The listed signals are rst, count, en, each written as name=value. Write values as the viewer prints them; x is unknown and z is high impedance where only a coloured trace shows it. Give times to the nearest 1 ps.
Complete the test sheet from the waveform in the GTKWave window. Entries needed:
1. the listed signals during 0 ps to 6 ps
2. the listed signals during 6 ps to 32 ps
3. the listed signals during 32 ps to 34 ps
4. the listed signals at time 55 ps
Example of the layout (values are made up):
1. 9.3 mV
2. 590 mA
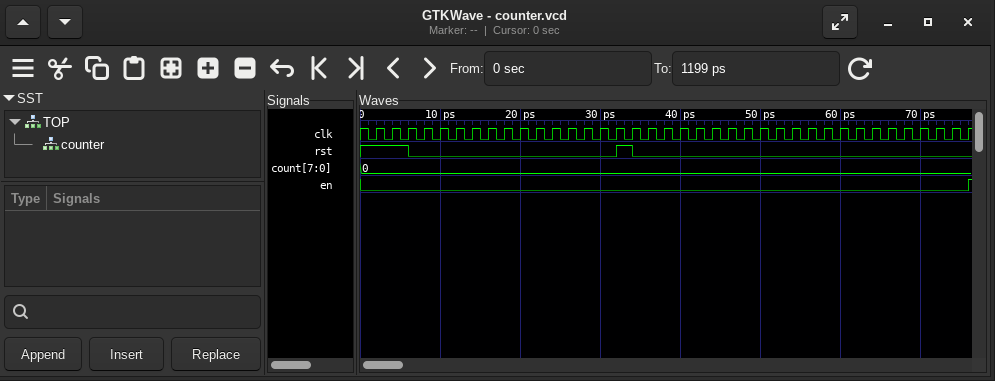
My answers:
1. rst=1, count=0, en=0
2. rst=0, count=0, en=0
3. rst=1, count=0, en=0
4. rst=0, count=0, en=0
